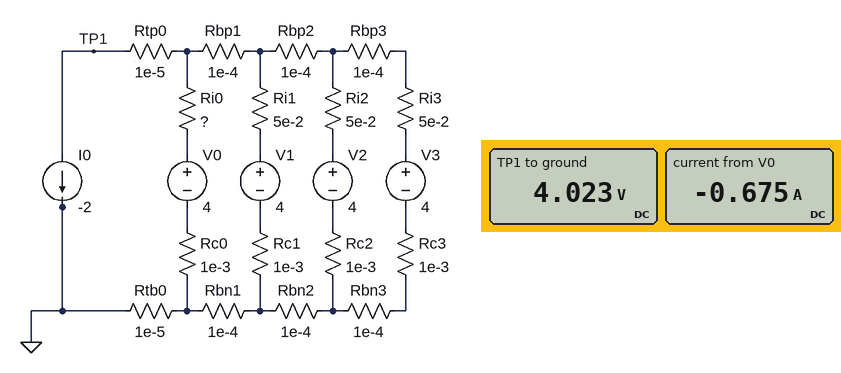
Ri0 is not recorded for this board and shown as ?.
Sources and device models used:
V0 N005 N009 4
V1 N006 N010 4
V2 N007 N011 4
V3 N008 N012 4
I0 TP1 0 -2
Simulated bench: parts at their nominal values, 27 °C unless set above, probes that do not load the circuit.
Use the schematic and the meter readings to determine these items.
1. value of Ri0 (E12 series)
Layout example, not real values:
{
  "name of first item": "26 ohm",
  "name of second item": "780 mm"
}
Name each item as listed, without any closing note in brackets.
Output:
{
  "value of Ri0": "0.033 Ω"
}
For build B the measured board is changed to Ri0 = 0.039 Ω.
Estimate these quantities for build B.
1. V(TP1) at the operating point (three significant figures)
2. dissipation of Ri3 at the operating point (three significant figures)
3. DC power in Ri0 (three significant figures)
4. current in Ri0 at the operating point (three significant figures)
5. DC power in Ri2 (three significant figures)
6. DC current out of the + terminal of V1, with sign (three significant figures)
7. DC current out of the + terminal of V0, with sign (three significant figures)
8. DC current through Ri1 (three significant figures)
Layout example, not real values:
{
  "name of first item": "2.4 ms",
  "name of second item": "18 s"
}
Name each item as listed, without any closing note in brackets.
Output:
{
  "V(TP1) at the operating point": "4.02 V",
  "dissipation of Ri3 at the operating point": "10.7 mW",
  "DC power in Ri0": "14.2 mW",
  "current in Ri0 at the operating point": "604 mA",
  "DC power in Ri2": "10.8 mW",
  "DC current out of the + terminal of V1, with sign": "-468 mA",
  "DC current out of the + terminal of V0, with sign": "-604 mA",
  "DC current through Ri1": "468 mA"
}
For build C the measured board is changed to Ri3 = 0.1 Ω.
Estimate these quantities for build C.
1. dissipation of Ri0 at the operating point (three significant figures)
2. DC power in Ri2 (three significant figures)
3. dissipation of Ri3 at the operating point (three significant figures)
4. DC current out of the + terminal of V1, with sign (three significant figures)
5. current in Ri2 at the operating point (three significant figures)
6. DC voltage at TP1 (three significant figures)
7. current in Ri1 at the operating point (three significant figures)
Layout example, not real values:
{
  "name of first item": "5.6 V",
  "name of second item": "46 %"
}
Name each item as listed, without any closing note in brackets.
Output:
{
  "dissipation of Ri0 at the operating point": "18.8 mW",
  "DC power in Ri2": "12.3 mW",
  "dissipation of Ri3 at the operating point": "6.24 mW",
  "DC current out of the + terminal of V1, with sign": "-499 mA",
  "current in Ri2 at the operating point": "496 mA",
  "DC voltage at TP1": "4.03 V",
  "current in Ri1 at the operating point": "499 mA"
}
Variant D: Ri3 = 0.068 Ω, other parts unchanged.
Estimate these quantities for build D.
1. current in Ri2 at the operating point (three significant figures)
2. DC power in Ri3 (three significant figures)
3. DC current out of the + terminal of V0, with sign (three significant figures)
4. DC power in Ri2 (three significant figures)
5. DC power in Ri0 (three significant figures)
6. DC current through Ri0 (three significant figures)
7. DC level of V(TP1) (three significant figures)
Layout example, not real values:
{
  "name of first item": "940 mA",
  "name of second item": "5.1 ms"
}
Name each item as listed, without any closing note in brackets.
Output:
{
  "current in Ri2 at the operating point": "468 mA",
  "DC power in Ri3": "8.10 mW",
  "DC current out of the + terminal of V0, with sign": "-715 mA",
  "DC power in Ri2": "11.0 mW",
  "DC power in Ri0": "16.9 mW",
  "DC current through Ri0": "715 mA",
  "DC level of V(TP1)": "4.02 V"
}
